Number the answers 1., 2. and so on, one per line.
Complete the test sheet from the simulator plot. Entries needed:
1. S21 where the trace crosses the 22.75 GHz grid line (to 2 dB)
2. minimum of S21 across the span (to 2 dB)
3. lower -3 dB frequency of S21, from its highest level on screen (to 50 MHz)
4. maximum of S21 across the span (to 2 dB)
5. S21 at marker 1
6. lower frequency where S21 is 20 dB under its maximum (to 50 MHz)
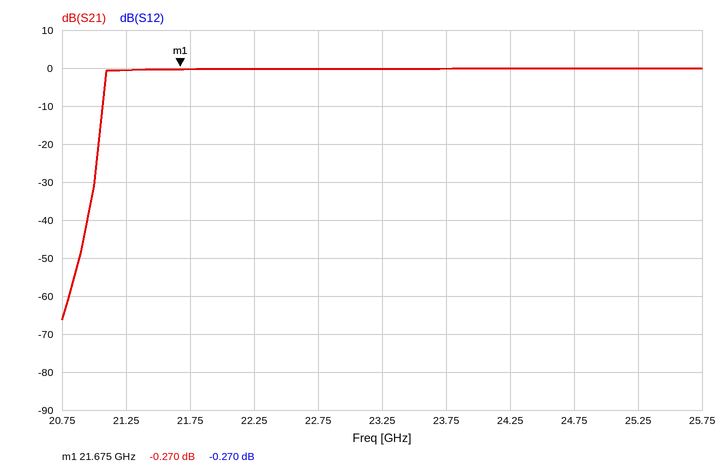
1. 0 dB
2. -66 dB
3. 21.10 GHz
4. 0 dB
5. -0.270 dB
6. 21.05 GHz
